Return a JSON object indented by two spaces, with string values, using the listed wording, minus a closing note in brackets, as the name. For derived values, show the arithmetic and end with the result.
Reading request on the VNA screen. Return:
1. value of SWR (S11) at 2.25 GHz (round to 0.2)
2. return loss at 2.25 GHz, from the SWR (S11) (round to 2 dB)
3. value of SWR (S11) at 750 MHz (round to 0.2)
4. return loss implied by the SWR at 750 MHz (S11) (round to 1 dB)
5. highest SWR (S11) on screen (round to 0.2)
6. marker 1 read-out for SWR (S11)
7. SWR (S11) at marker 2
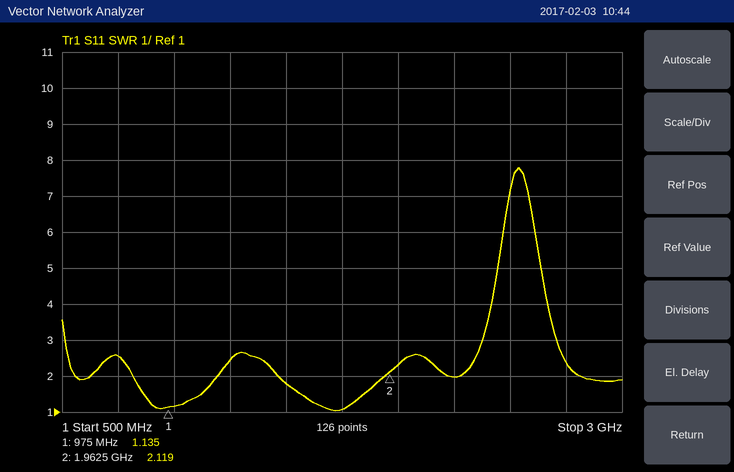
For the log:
{
  "value of SWR (S11) at 2.25 GHz": "2.0",
  "return loss at 2.25 GHz, from the SWR (S11)": "−20 log10((2 − 1)/(2 + 1)) ≈ 10 dB",
  "value of SWR (S11) at 750 MHz": "2.6",
  "return loss implied by the SWR at 750 MHz (S11)": "−20 log10((2.6 − 1)/(2.6 + 1)) ≈ 7 dB",
  "highest SWR (S11) on screen": "7.8",
  "marker 1 read-out for SWR": "1.135",
  "SWR (S11) at marker 2": "2.119"
}
